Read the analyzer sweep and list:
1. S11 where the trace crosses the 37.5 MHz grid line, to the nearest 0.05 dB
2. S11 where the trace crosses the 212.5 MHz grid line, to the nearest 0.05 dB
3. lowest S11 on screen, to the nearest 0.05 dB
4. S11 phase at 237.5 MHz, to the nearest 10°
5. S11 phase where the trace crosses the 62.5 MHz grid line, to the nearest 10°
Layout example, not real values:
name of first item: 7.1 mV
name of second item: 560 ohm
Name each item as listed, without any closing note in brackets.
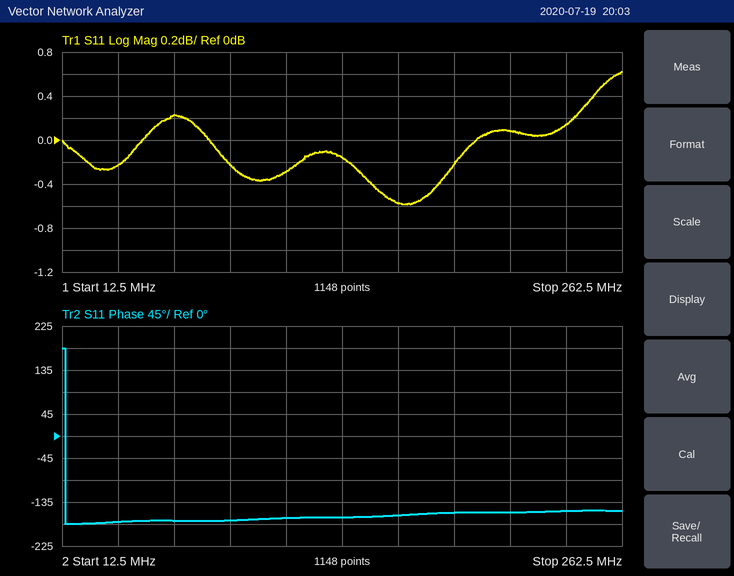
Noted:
S11 where the trace crosses the 37.5 MHz grid line, to the nearest 0.05 dB: -0.25 dB
S11 where the trace crosses the 212.5 MHz grid line, to the nearest 0.05 dB: 0.10 dB
lowest S11 on screen, to the nearest 0.05 dB: -0.60 dB
S11 phase at 237.5 MHz, to the nearest 10°: -150°
S11 phase where the trace crosses the 62.5 MHz grid line, to the nearest 10°: -170°
